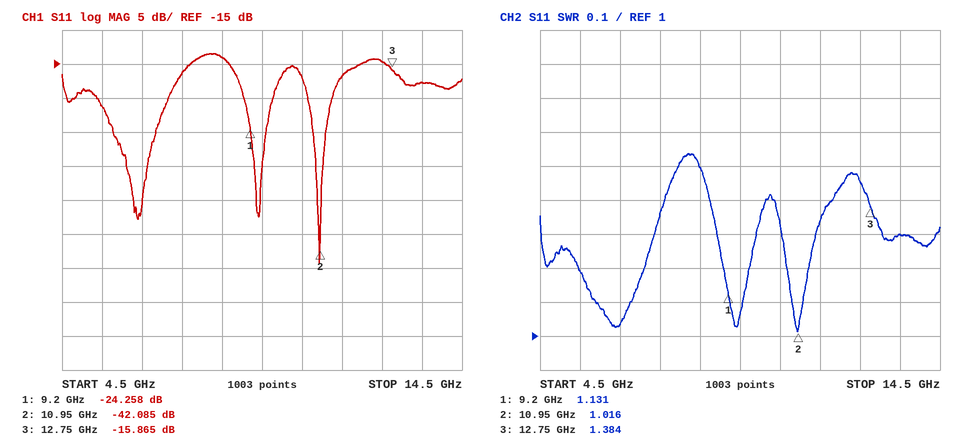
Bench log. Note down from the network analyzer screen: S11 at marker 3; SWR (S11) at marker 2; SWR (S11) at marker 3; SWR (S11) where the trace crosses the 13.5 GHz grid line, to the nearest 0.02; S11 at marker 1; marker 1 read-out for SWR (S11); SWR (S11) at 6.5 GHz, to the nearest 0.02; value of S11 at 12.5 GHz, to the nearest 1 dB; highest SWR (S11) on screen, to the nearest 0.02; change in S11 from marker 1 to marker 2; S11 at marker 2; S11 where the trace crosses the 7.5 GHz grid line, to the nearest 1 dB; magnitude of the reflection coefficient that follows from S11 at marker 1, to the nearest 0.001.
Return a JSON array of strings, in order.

["-15.865 dB", "1.016", "1.384", "1.30", "-24.258 dB", "1.131", "1.04", "-15 dB", "1.54", "-17.827 dB", "-42.085 dB", "-16 dB", "0.061"]
